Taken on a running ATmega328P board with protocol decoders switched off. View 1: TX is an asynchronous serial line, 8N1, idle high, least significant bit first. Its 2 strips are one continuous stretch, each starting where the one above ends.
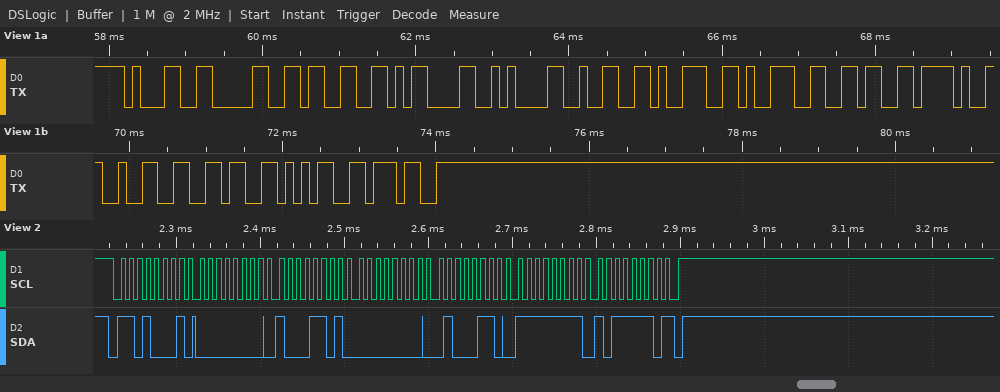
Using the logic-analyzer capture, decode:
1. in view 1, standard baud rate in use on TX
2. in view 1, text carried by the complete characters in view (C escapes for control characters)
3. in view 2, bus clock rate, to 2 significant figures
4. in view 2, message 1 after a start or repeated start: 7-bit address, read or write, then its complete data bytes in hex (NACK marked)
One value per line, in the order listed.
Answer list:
9600 baud
"103\r\n2996/2657"
100 kHz
0x68 read: 00 8D 00 46 FF BE NACK
